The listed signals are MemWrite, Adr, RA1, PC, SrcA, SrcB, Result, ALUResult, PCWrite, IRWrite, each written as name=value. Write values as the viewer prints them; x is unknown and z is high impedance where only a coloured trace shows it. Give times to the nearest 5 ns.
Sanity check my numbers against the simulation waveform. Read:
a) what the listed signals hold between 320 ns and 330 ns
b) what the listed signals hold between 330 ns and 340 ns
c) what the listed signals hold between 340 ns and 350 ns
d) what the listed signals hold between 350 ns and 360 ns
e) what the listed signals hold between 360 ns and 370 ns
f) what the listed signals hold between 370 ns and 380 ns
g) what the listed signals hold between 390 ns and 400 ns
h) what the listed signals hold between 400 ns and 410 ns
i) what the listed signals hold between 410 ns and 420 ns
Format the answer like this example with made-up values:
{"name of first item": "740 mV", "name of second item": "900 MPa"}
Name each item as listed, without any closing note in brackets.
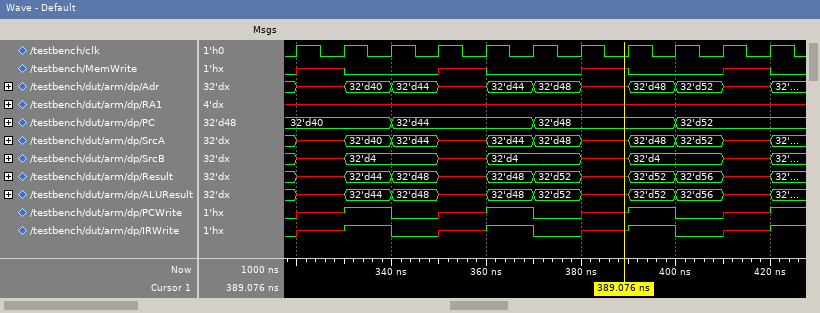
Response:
{"what the listed signals hold between 320 ns and 330 ns": "MemWrite=x, Adr=x, RA1=x, PC=32'd40, SrcA=x, SrcB=x, Result=x, ALUResult=x, PCWrite=x, IRWrite=x", "what the listed signals hold between 330 ns and 340 ns": "MemWrite=0, Adr=32'd40, RA1=x, PC=32'd40, SrcA=32'd40, SrcB=32'd4, Result=32'd44, ALUResult=32'd44, PCWrite=1, IRWrite=1", "what the listed signals hold between 340 ns and 350 ns": "MemWrite=0, Adr=32'd44, RA1=x, PC=32'd44, SrcA=32'd44, SrcB=32'd4, Result=32'd48, ALUResult=32'd48, PCWrite=0, IRWrite=0", "what the listed signals hold between 350 ns and 360 ns": "MemWrite=x, Adr=x, RA1=x, PC=32'd44, SrcA=x, SrcB=x, Result=x, ALUResult=x, PCWrite=x, IRWrite=x", "what the listed signals hold between 360 ns and 370 ns": "MemWrite=0, Adr=32'd44, RA1=x, PC=32'd44, SrcA=32'd44, SrcB=32'd4, Result=32'd48, ALUResult=32'd48, PCWrite=1, IRWrite=1", "what the listed signals hold between 370 ns and 380 ns": "MemWrite=0, Adr=32'd48, RA1=x, PC=32'd48, SrcA=32'd48, SrcB=32'd4, Result=32'd52, ALUResult=32'd52, PCWrite=0, IRWrite=0", "what the listed signals hold between 390 ns and 400 ns": "MemWrite=0, Adr=32'd48, RA1=x, PC=32'd48, SrcA=32'd48, SrcB=32'd4, Result=32'd52, ALUResult=32'd52, PCWrite=1, IRWrite=1", "what the listed signals hold between 400 ns and 410 ns": "MemWrite=0, Adr=32'd52, RA1=x, PC=32'd52, SrcA=32'd52, SrcB=32'd4, Result=32'd56, ALUResult=32'd56, PCWrite=0, IRWrite=0", "what the listed signals hold between 410 ns and 420 ns": "MemWrite=x, Adr=x, RA1=x, PC=32'd52, SrcA=x, SrcB=x, Result=x, ALUResult=x, PCWrite=x, IRWrite=x"}
